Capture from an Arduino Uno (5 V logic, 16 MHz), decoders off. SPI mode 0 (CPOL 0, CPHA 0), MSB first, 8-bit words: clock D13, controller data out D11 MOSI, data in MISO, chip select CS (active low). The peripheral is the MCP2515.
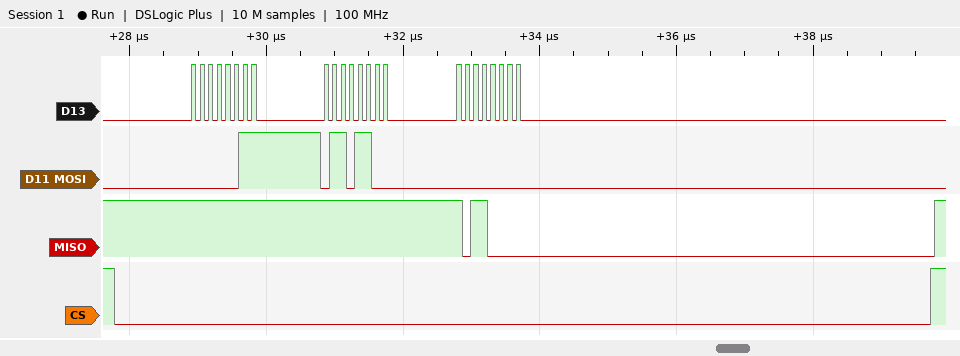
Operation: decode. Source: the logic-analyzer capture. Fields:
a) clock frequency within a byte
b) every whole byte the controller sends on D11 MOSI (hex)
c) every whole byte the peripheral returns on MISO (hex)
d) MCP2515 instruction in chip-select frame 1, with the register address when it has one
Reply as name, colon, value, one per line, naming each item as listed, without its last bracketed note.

clock frequency within a byte: 8 MHz
every whole byte the controller sends on D11 MOSI: 0x03 0x6C 0x00
every whole byte the peripheral returns on MISO: 0xFF 0xFF 0xB0
MCP2515 instruction in chip-select frame 1, with the register address when it has one: READ 0x6C
